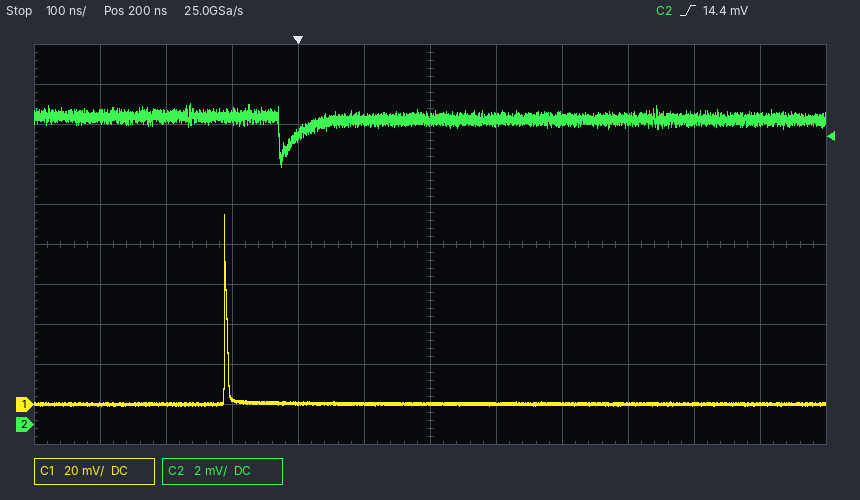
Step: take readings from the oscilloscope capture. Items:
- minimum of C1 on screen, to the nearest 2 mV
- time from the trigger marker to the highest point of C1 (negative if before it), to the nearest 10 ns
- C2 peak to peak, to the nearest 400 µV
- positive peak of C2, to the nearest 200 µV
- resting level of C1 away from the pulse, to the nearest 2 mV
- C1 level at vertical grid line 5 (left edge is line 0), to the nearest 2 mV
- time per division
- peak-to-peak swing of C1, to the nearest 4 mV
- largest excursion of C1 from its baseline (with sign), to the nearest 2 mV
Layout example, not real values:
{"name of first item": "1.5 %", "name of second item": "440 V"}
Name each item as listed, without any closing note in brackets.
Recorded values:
{"minimum of C1 on screen, to the nearest 2 mV": "0 mV", "time from the trigger marker to the highest point of C1 (negative if before it), to the nearest 10 ns": "-110 ns", "C2 peak to peak, to the nearest 400 µV": "3.2 mV", "positive peak of C2, to the nearest 200 µV": "16.0 mV", "resting level of C1 away from the pulse, to the nearest 2 mV": "0 mV", "C1 level at vertical grid line 5 (left edge is line 0), to the nearest 2 mV": "0 mV", "time per division": "100 ns", "peak-to-peak swing of C1, to the nearest 4 mV": "96 mV", "largest excursion of C1 from its baseline (with sign), to the nearest 2 mV": "+94 mV"}
